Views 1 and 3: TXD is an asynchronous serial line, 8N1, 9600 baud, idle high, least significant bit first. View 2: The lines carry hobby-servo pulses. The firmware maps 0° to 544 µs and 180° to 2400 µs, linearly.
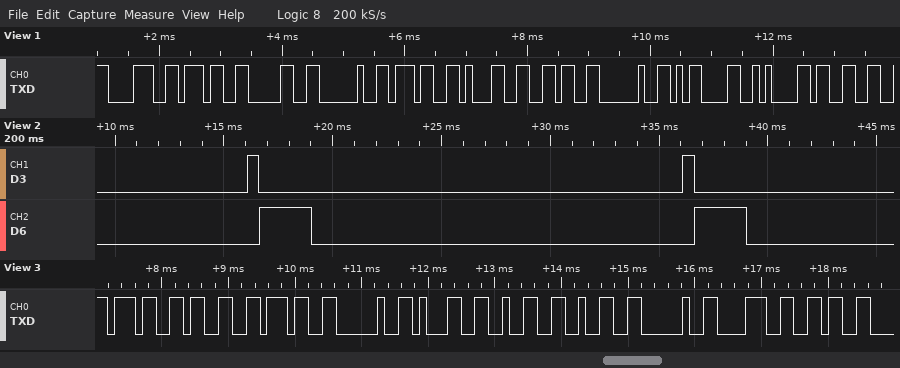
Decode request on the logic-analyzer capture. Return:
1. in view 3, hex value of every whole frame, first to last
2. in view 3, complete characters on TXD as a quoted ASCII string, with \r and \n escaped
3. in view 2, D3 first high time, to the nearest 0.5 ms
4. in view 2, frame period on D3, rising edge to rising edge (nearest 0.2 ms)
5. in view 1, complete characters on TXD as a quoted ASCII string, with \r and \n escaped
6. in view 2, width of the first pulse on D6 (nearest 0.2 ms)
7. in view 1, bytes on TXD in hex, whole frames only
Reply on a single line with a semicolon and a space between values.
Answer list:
37 33 37 20 31 32 32 20 38 36; "737 122 86"; 0.5 ms; 20.0 ms; "870 716 \r\n3"; 2.4 ms; 38 37 30 20 37 31 36 20 0D 0A 33
